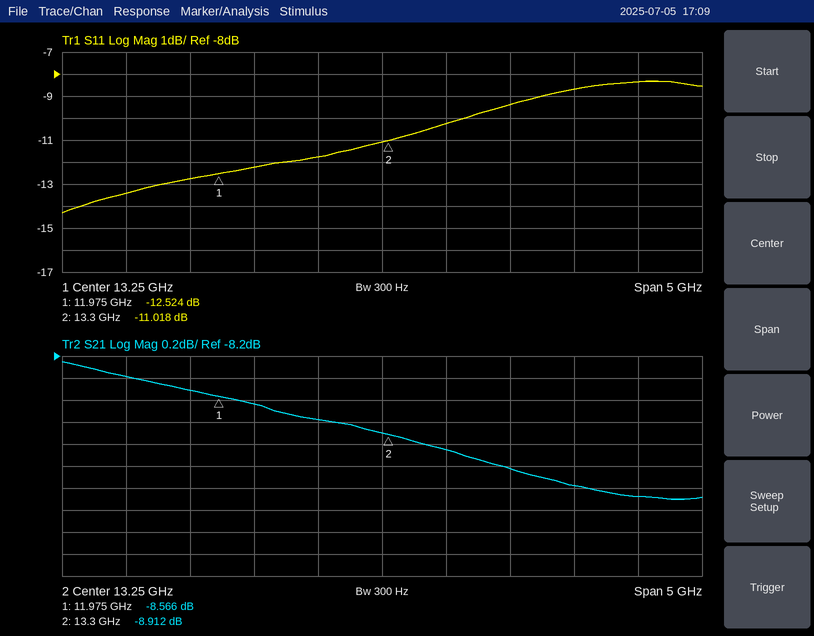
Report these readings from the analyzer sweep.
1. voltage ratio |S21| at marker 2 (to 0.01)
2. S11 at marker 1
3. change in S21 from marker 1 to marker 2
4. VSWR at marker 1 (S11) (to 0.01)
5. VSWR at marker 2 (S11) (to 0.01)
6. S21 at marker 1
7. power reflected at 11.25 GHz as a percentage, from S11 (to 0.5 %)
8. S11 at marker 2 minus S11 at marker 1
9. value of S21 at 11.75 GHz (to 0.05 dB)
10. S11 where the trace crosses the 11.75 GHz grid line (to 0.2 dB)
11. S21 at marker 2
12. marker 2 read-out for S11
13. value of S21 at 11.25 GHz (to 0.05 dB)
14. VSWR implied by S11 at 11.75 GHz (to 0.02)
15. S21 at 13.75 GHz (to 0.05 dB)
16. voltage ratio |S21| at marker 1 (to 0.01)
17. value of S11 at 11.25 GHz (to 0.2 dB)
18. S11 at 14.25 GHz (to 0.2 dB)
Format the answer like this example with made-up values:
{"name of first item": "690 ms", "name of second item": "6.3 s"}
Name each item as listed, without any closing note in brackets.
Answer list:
{"voltage ratio |S21| at marker 2": "0.36", "S11 at marker 1": "-12.524 dB", "change in S21 from marker 1 to marker 2": "-0.346 dB", "VSWR at marker 1 (S11)": "1.62", "VSWR at marker 2 (S11)": "1.78", "S21 at marker 1": "-8.566 dB", "power reflected at 11.25 GHz as a percentage, from S11": "4.5 %", "S11 at marker 2 minus S11 at marker 1": "1.506 dB", "value of S21 at 11.75 GHz": "-8.50 dB", "S11 where the trace crosses the 11.75 GHz grid line": "-12.8 dB", "S21 at marker 2": "-8.912 dB", "marker 2 read-out for S11": "-11.018 dB", "value of S21 at 11.25 GHz": "-8.40 dB", "VSWR implied by S11 at 11.75 GHz": "1.60", "S21 at 13.75 GHz": "-9.05 dB", "voltage ratio |S21| at marker 1": "0.37", "value of S11 at 11.25 GHz": "-13.4 dB", "S11 at 14.25 GHz": "-9.4 dB"}
